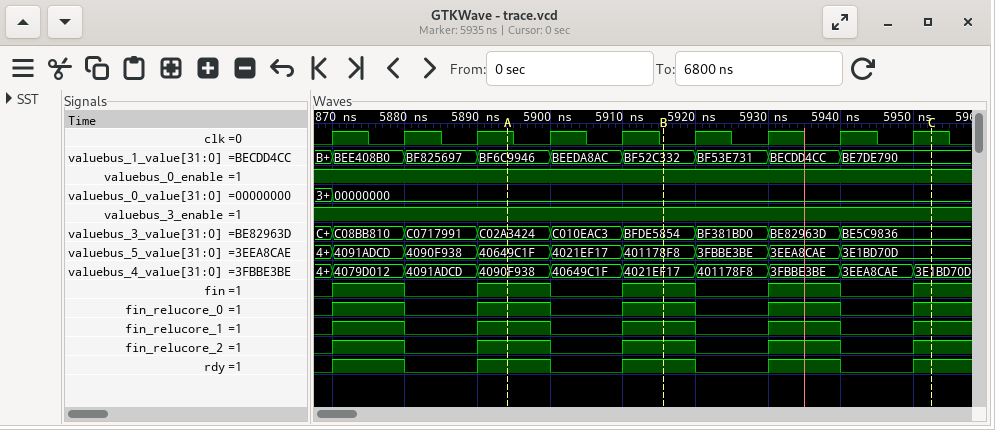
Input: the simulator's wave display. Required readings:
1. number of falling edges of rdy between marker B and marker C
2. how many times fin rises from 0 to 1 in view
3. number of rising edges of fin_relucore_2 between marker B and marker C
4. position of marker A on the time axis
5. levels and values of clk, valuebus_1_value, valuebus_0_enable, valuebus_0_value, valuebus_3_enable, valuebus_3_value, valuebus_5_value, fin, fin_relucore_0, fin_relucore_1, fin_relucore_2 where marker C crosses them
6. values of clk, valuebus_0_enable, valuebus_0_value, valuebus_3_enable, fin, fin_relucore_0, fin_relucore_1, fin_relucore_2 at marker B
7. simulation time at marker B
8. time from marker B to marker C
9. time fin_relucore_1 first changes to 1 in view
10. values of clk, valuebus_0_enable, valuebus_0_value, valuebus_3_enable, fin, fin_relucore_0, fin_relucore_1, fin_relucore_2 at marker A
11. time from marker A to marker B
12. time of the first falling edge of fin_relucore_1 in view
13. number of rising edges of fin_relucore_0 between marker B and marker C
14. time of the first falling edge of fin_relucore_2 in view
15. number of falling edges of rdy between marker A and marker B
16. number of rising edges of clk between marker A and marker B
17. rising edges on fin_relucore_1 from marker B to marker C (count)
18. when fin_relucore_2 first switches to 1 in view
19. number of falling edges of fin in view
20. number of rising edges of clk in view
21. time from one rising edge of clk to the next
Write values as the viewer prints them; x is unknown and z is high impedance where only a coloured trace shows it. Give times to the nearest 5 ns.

2
5
2
5895 ns
clk=1, valuebus_1_value=BE7DE790, valuebus_0_enable=1, valuebus_0_value=00000000, valuebus_3_enable=1, valuebus_3_value=BE5C9836, valuebus_5_value=3E1BD70D, fin=1, fin_relucore_0=1, fin_relucore_1=1, fin_relucore_2=1
clk=0, valuebus_0_enable=1, valuebus_0_value=00000000, valuebus_3_enable=1, fin=1, fin_relucore_0=1, fin_relucore_1=1, fin_relucore_2=1
5915 ns
35 ns
5870 ns
clk=1, valuebus_0_enable=1, valuebus_0_value=00000000, valuebus_3_enable=1, fin=1, fin_relucore_0=1, fin_relucore_1=1, fin_relucore_2=1
20 ns
5880 ns
2
5880 ns
1
2
2
5870 ns
4
9
10 ns
